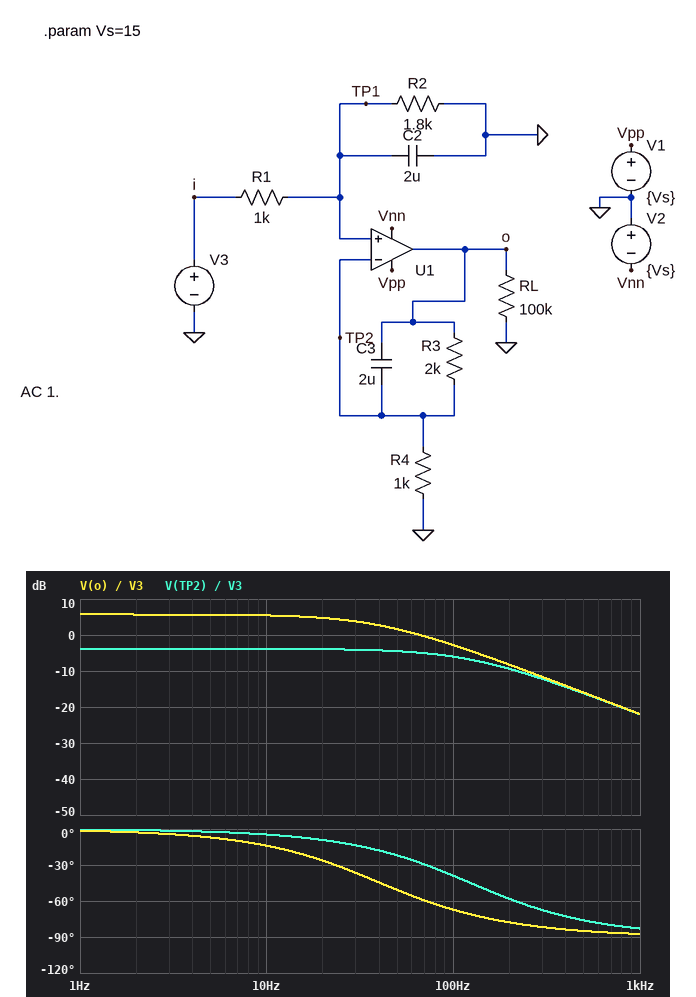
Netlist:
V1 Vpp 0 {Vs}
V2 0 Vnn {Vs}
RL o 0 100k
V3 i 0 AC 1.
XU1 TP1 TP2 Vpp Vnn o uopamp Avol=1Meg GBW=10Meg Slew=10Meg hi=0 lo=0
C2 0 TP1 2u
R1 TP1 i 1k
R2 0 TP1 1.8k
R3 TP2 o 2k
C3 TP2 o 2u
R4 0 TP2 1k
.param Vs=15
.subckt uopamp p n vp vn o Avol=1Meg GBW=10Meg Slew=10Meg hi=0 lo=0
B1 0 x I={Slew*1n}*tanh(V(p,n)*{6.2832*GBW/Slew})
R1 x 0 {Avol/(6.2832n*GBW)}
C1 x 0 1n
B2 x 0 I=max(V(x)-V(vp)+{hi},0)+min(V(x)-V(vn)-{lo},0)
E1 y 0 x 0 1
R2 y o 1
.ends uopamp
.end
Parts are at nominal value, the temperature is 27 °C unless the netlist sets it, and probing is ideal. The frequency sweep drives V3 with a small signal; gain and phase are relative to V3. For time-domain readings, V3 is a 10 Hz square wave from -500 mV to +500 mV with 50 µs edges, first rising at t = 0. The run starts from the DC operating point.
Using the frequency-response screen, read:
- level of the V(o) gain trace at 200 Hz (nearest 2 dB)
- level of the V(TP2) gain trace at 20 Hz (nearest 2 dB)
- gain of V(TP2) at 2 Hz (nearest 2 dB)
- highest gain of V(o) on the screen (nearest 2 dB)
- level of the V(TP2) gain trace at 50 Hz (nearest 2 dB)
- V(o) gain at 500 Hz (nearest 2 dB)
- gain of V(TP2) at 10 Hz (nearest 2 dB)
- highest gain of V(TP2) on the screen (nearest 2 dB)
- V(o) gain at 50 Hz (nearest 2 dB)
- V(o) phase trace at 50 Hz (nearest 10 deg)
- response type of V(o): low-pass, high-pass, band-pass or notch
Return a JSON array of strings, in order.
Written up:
["-8 dB", "-4 dB", "-4 dB", "6 dB", "-4 dB", "-16 dB", "-4 dB", "-4 dB", "2 dB", "-50 deg", "low-pass"]
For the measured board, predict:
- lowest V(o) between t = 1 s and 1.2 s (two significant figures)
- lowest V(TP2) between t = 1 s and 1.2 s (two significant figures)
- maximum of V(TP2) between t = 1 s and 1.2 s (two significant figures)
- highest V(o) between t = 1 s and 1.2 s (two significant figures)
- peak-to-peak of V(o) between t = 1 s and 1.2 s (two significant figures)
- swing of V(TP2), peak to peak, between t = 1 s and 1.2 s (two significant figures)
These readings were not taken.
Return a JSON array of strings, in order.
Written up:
["-960 mV", "-320 mV", "320 mV", "960 mV", "1.9 V", "640 mV"]
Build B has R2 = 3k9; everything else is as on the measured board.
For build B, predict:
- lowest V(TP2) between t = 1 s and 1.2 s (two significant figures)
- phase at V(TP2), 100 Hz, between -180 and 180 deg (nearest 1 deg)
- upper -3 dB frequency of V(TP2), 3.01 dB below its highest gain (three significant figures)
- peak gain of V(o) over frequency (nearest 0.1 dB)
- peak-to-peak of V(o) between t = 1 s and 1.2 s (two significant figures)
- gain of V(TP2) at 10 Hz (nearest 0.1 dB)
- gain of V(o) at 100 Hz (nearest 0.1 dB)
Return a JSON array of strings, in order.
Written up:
["-400 mV", "-45 deg", "100 Hz", "7.6 dB", "2.4 V", "-2.0 dB", "-1.8 dB"]
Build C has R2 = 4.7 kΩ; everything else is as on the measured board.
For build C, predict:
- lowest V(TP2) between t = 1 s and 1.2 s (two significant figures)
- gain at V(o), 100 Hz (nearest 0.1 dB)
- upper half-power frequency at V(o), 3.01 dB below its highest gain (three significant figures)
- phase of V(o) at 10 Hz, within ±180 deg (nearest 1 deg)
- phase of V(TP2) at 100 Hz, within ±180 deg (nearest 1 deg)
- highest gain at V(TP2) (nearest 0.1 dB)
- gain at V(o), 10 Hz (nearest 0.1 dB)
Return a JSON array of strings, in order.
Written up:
["-410 mV", "-1.6 dB", "37.9 Hz", "-15 deg", "-46 deg", "-1.7 dB", "7.6 dB"]
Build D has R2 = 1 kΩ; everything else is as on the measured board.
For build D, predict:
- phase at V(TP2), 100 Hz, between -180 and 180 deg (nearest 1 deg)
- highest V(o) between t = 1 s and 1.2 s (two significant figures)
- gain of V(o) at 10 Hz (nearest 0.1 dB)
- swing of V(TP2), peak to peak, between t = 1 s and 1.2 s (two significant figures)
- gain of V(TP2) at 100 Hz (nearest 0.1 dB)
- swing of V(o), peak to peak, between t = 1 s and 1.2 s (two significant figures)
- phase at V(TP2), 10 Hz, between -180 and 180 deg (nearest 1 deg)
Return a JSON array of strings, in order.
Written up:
["-32 deg", "750 mV", "3.3 dB", "500 mV", "-7.5 dB", "1.5 V", "-4 deg"]
